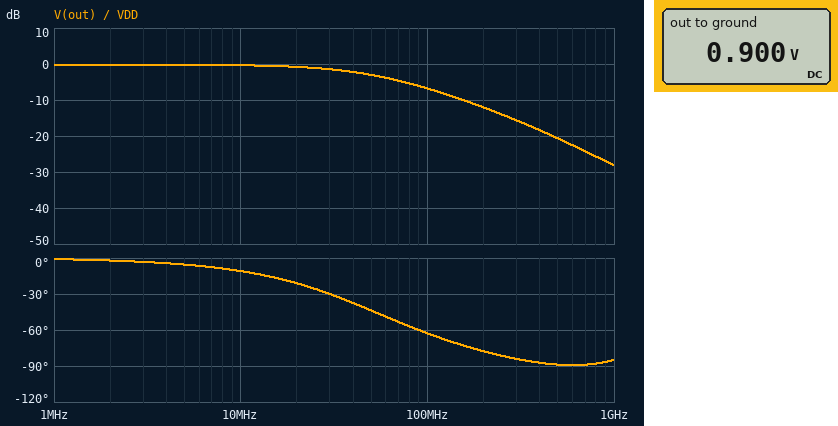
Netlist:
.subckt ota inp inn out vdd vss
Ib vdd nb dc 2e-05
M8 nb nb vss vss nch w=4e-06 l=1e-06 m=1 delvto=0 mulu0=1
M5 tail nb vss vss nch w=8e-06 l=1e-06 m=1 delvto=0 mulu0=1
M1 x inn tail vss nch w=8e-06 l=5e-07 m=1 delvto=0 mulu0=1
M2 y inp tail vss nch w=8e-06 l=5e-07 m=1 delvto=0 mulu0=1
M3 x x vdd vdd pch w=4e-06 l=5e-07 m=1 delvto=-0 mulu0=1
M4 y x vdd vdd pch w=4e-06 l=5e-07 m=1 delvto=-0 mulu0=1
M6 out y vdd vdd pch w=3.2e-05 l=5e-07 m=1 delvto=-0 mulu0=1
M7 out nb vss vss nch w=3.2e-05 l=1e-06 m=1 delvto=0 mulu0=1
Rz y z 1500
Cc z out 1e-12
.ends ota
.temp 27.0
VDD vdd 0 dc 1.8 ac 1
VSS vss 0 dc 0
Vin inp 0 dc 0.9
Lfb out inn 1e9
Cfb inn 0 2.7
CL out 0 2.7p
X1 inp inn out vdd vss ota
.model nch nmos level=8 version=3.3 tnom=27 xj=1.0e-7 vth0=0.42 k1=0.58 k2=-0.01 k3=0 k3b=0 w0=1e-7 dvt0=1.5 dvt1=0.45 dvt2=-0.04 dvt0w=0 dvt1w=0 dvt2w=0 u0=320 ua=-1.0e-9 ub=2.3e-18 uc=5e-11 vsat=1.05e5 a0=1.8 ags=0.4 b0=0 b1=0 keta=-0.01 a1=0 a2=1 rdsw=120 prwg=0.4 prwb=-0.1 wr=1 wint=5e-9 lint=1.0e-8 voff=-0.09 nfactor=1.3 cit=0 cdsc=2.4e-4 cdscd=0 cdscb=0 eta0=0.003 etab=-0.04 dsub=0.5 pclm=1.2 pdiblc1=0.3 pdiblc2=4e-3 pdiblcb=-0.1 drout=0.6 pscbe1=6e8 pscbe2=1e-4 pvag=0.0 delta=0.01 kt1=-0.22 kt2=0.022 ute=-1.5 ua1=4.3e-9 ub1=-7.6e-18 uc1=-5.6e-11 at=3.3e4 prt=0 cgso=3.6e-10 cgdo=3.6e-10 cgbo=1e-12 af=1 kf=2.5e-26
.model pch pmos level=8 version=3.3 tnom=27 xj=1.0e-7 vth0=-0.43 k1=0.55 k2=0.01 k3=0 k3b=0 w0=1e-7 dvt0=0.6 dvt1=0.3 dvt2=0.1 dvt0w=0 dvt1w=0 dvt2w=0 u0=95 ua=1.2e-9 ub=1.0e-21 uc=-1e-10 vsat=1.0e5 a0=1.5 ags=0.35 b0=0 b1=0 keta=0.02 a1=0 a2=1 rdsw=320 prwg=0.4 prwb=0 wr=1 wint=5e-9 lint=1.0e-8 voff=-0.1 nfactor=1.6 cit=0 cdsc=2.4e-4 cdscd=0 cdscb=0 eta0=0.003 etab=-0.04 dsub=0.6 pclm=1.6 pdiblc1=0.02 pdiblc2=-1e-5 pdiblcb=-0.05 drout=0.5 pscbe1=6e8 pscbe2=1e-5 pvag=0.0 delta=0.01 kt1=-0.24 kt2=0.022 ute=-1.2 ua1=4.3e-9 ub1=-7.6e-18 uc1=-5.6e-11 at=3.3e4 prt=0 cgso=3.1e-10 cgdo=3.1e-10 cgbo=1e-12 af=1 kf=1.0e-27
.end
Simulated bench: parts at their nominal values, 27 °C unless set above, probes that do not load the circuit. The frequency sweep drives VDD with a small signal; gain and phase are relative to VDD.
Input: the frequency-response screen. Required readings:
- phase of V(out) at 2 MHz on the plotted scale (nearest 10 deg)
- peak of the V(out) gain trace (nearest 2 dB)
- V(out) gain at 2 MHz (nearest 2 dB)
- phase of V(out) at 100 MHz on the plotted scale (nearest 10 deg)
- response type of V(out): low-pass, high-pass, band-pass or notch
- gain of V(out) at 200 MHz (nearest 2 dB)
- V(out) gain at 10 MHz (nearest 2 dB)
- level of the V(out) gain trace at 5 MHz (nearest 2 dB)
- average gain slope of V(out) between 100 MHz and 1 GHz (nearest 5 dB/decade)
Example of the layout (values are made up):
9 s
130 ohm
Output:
0 deg
0 dB
0 dB
-60 deg
low-pass
-12 dB
0 dB
0 dB
-20 dB/decade
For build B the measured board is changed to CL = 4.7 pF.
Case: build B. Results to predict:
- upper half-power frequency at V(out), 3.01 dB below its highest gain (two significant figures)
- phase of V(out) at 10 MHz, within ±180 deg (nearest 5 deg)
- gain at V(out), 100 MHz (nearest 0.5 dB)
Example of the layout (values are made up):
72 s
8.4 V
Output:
31 MHz
-20 deg
-11.0 dB
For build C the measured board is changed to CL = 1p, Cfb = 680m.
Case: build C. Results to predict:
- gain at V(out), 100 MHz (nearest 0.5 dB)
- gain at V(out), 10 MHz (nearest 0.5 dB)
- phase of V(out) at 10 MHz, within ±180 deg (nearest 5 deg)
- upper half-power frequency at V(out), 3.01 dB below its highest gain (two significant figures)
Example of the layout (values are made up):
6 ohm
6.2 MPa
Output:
-2.0 dB
0 dB
-5 deg
130 MHz
